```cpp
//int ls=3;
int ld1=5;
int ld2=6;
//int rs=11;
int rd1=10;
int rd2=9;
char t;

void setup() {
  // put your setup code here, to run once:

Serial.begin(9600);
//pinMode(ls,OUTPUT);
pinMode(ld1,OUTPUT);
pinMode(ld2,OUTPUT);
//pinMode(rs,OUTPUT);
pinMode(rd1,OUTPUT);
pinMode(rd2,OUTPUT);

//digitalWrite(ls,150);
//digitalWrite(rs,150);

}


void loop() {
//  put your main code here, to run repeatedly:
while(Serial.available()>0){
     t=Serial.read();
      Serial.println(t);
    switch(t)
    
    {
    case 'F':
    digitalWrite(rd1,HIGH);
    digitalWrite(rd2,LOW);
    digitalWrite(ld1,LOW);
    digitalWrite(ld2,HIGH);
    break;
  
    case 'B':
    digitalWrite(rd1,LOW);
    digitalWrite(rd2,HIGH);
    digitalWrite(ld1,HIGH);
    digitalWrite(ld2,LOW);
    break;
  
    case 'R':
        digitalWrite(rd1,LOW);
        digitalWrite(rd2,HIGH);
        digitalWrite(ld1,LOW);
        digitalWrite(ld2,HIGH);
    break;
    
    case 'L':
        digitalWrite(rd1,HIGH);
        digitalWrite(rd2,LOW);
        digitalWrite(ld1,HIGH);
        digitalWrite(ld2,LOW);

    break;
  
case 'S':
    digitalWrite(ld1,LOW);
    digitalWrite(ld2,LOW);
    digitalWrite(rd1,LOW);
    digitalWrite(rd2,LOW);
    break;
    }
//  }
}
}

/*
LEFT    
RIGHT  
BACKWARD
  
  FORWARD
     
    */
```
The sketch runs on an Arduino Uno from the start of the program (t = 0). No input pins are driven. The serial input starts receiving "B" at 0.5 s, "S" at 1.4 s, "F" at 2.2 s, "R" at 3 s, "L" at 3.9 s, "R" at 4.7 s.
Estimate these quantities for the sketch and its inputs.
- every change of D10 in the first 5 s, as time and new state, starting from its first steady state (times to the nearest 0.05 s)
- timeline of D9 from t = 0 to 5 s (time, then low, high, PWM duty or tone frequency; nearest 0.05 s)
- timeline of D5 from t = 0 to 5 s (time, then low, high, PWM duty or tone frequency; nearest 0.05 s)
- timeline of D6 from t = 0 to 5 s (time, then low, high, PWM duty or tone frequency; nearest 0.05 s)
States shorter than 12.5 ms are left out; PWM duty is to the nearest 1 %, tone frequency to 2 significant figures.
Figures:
0 s low; 2.2 s high; 3 s low; 3.9 s high; 4.7 s low
0 s low; 0.5 s high; 1.4 s low; 3 s high; 3.9 s low; 4.7 s high
0 s low; 0.5 s high; 1.4 s low; 3.9 s high; 4.7 s low
0 s low; 2.2 s high; 3.9 s low; 4.7 s high
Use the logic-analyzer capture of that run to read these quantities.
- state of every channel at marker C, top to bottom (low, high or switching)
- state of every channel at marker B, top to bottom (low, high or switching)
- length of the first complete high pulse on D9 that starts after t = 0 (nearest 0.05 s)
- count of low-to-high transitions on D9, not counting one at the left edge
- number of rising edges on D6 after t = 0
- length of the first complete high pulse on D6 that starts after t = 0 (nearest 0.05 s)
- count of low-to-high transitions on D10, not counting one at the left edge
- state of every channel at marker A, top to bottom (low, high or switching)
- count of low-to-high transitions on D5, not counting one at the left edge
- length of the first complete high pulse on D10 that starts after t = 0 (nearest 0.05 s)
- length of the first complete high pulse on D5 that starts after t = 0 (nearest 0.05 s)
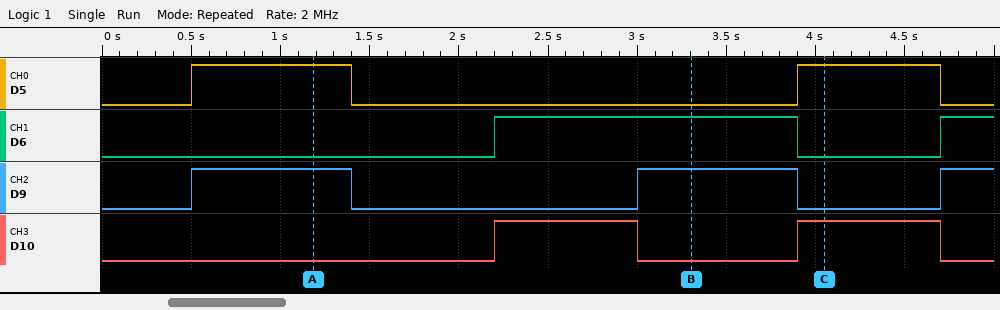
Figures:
D5 high, D6 low, D9 low, D10 high
D5 low, D6 high, D9 high, D10 low
0.90 s
3
2
1.70 s
2
D5 high, D6 low, D9 high, D10 low
2
0.80 s
0.90 s
